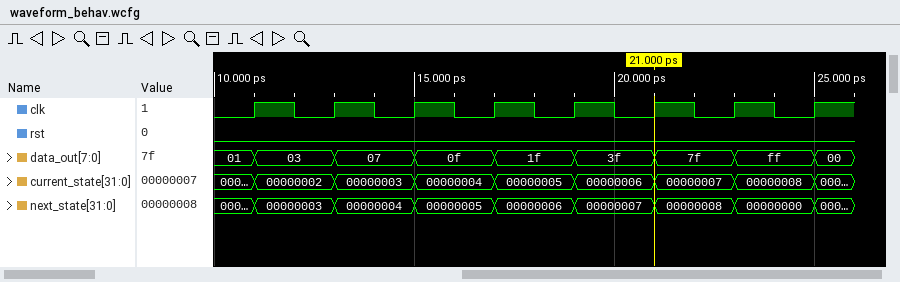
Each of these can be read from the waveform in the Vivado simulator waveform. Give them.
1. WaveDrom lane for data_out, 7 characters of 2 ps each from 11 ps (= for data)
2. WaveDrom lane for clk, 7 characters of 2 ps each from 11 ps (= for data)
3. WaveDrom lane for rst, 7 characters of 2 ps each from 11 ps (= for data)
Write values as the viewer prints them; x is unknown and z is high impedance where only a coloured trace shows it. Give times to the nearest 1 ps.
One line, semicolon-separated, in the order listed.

{name: 'data_out', wave: '=======', data: '03 07 0f 1f 3f 7f ff'}; {name: 'clk', wave: 'p......'}; {name: 'rst', wave: '0......'}
